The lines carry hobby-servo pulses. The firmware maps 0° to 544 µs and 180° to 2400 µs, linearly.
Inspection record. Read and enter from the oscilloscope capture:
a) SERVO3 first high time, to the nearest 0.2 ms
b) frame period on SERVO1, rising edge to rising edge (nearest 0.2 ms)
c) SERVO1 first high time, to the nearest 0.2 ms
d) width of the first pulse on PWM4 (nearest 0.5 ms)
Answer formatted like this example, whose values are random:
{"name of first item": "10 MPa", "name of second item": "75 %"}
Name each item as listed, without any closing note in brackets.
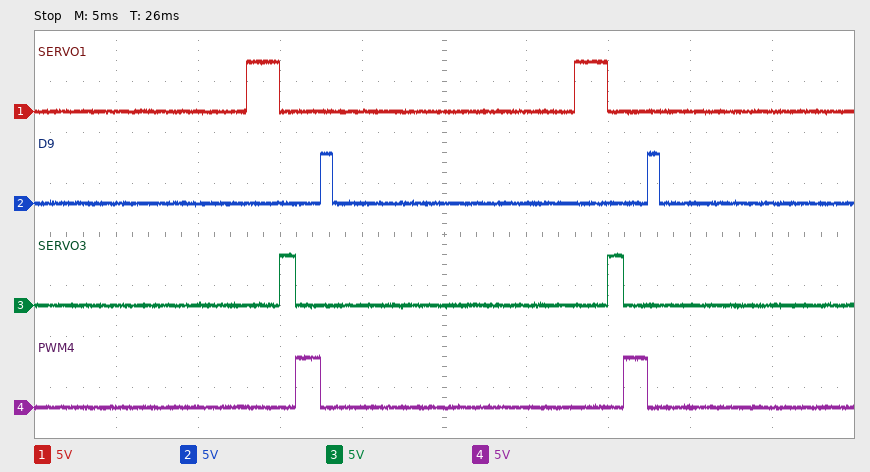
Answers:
{"SERVO3 first high time, to the nearest 0.2 ms": "1.0 ms", "frame period on SERVO1, rising edge to rising edge": "20.0 ms", "SERVO1 first high time, to the nearest 0.2 ms": "2.0 ms", "width of the first pulse on PWM4": "1.5 ms"}
